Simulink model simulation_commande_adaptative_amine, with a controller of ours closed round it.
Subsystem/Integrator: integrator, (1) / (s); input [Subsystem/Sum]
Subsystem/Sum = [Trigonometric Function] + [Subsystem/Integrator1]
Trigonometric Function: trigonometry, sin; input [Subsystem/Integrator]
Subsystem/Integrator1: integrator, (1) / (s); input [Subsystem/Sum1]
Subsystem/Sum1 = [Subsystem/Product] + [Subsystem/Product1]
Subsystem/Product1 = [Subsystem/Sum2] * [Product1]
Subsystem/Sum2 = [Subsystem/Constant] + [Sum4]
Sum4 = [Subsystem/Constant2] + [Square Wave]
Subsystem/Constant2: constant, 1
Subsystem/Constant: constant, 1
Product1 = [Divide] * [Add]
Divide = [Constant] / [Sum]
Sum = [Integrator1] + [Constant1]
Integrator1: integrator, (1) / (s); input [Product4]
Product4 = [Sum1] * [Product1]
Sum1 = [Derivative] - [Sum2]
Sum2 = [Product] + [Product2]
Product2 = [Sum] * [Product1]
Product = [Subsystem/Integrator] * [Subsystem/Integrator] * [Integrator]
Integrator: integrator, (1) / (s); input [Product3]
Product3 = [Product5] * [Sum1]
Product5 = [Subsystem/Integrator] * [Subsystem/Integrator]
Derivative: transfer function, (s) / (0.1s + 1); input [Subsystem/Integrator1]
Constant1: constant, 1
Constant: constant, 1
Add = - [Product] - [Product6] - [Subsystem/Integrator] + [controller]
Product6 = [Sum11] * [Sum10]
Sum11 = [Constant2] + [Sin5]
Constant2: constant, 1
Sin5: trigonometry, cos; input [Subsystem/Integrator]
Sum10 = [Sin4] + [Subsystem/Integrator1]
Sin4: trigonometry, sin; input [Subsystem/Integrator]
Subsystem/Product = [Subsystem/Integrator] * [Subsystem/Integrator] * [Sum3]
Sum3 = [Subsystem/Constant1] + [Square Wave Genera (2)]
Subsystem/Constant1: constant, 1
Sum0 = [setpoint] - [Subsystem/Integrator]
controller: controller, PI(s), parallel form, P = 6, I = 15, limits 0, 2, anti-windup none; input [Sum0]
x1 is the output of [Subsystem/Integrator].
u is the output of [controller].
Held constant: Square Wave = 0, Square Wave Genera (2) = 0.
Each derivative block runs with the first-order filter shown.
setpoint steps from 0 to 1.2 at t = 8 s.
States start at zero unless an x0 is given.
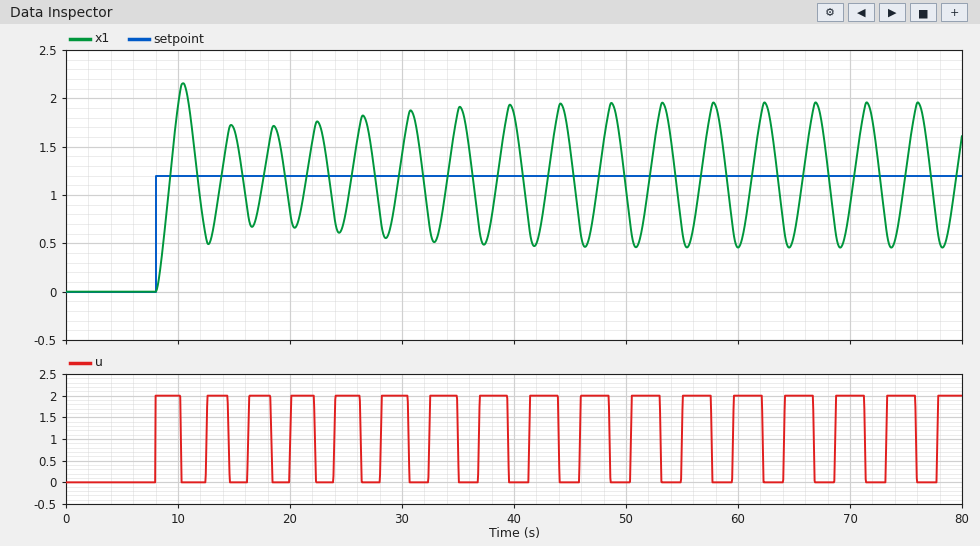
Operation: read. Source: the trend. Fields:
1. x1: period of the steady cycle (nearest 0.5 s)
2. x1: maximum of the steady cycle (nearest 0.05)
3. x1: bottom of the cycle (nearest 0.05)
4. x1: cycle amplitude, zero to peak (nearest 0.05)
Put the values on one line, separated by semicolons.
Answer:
4.5 s; 1.95; 0.45; 0.75
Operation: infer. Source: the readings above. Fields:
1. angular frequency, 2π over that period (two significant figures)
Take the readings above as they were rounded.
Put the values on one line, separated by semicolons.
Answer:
1.4 rad/s
